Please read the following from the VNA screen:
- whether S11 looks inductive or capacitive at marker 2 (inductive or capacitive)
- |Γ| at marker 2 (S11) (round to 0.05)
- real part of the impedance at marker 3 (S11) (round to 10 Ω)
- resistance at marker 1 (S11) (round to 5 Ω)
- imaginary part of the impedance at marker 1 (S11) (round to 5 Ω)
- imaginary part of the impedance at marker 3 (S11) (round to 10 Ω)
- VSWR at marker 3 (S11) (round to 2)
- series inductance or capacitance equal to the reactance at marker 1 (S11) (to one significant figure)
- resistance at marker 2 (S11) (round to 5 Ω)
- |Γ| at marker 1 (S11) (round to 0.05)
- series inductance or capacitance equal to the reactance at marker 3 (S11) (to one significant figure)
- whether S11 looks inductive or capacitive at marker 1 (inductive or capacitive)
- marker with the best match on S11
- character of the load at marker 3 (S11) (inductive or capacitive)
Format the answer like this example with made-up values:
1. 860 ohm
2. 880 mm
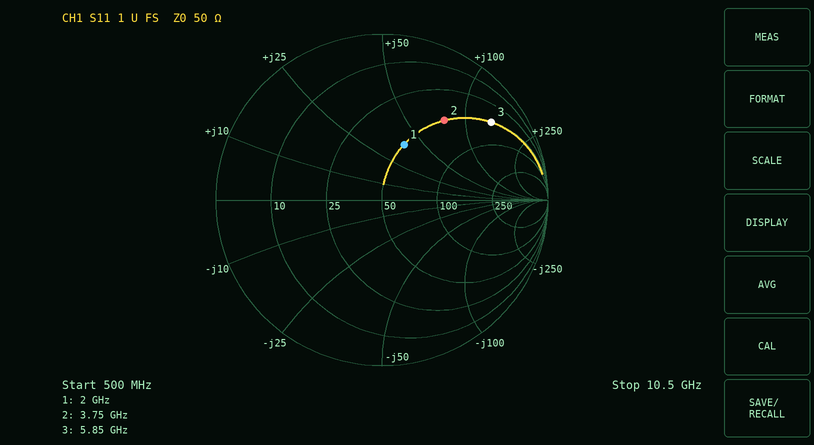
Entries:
1. inductive
2. 0.60
3. 50 Ω
4. 50 Ω
5. +40 Ω
6. +140 Ω
7. 10
8. 3 nH
9. 50 Ω
10. 0.35
11. 4 nH
12. inductive
13. marker 1
14. inductive
